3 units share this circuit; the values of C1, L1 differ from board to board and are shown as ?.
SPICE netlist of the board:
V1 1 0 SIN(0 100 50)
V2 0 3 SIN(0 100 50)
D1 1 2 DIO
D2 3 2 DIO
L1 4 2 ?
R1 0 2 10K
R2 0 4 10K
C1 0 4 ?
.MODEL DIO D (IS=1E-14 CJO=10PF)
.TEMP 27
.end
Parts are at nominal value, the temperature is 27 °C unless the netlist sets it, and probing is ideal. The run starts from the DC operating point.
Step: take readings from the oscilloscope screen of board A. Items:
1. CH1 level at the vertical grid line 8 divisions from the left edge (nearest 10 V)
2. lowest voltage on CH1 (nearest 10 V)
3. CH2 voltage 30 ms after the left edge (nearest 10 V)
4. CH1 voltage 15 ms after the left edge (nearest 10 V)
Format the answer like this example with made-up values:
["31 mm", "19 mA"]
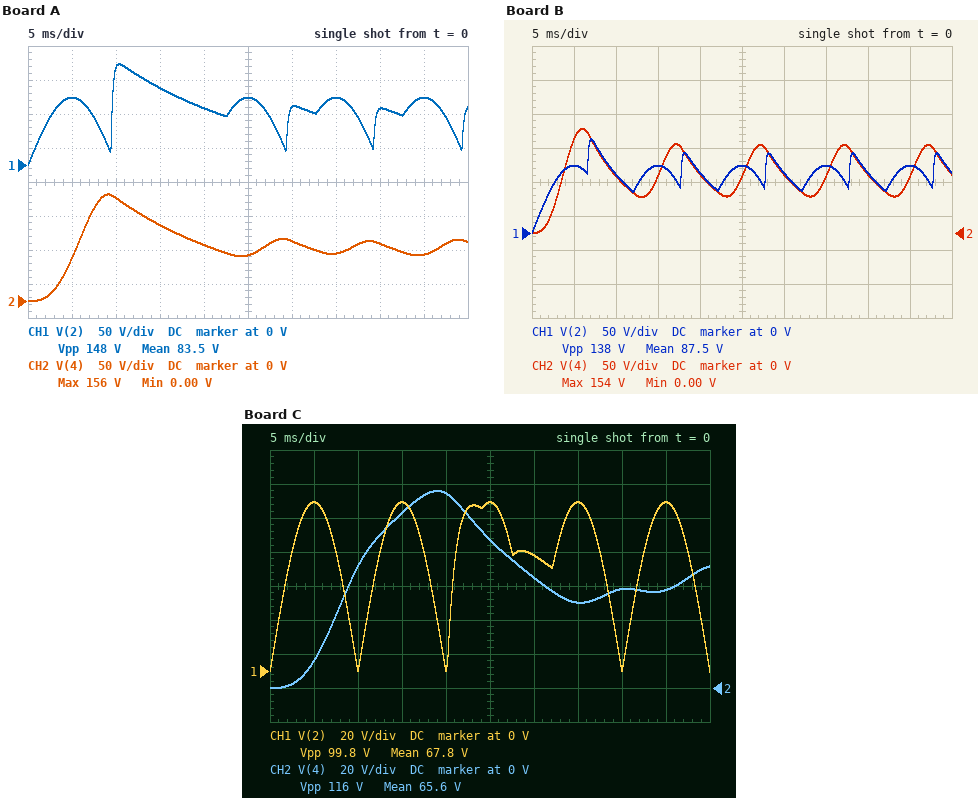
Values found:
["80 V", "0 V", "90 V", "110 V"]
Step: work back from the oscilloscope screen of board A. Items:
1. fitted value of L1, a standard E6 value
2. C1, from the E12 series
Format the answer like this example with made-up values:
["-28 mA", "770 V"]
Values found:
["2.2 H", "3.3 µF"]
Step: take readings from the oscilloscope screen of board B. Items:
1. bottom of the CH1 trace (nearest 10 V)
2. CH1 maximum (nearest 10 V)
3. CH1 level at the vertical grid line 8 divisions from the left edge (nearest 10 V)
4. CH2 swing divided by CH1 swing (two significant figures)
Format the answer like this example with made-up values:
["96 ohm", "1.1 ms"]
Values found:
["0 V", "140 V", "90 V", "1.1"]
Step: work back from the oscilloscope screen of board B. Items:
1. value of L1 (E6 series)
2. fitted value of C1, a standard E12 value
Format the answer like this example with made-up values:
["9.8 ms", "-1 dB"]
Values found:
["1.5 H", "1.2 µF"]
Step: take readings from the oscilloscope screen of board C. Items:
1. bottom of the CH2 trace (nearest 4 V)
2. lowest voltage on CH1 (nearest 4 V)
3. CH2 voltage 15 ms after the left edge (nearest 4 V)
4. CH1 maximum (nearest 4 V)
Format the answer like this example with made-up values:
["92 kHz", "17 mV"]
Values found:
["0 V", "0 V", "104 V", "100 V"]
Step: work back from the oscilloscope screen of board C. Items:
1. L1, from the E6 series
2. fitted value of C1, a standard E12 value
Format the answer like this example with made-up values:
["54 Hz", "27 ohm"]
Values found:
["10 H", "3.3 µF"]
